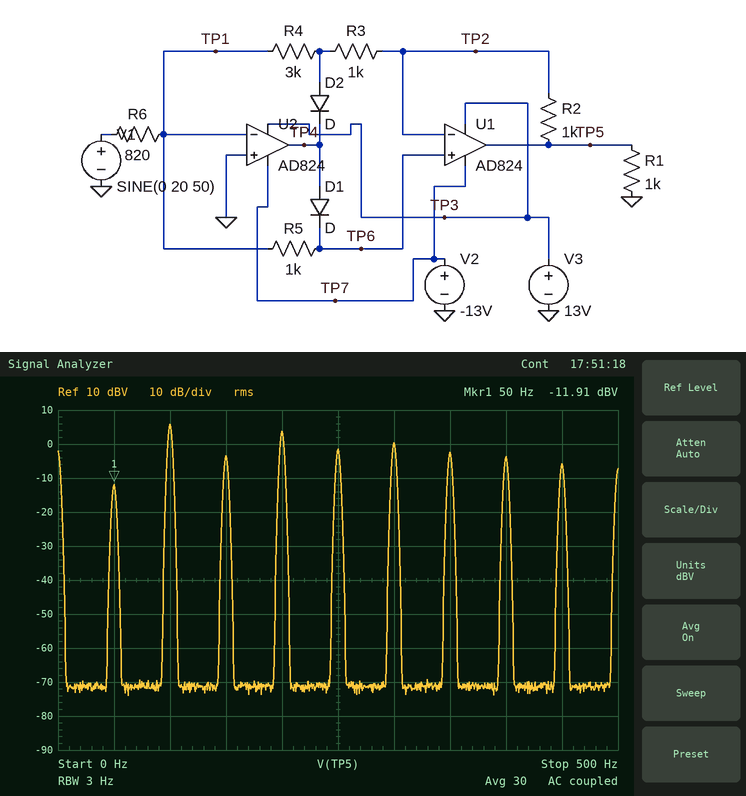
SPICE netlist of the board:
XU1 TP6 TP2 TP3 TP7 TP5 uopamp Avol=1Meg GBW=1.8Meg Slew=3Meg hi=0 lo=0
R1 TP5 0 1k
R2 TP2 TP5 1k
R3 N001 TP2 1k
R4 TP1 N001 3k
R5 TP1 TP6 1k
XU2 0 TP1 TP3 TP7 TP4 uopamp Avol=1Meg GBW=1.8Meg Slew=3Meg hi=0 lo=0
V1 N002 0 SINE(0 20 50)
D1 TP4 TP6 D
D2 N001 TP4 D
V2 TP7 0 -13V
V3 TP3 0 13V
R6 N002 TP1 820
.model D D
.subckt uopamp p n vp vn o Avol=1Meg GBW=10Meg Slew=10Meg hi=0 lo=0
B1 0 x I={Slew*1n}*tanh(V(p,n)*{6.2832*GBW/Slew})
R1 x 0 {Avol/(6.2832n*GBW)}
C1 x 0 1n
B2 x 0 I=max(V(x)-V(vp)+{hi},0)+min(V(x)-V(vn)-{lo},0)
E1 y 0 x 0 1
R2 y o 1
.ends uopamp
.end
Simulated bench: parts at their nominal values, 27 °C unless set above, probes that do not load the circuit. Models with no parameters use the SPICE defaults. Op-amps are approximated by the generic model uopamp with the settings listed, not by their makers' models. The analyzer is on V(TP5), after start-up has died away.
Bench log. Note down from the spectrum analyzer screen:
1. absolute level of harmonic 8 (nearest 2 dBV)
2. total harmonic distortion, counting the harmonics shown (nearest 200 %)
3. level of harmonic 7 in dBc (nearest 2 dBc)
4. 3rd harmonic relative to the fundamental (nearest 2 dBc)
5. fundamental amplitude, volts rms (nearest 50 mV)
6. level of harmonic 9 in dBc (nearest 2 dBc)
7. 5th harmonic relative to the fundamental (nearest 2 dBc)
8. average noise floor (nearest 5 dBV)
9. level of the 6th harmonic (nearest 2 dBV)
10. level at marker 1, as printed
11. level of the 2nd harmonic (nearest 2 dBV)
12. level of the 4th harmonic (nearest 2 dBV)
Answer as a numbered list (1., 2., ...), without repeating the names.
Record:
1. -4 dBV
2. 1200 %
3. 10 dBc
4. 8 dBc
5. 250 mV
6. 6 dBc
7. 10 dBc
8. -70 dBV
9. 0 dBV
10. -11.91 dBV
11. 6 dBV
12. 4 dBV
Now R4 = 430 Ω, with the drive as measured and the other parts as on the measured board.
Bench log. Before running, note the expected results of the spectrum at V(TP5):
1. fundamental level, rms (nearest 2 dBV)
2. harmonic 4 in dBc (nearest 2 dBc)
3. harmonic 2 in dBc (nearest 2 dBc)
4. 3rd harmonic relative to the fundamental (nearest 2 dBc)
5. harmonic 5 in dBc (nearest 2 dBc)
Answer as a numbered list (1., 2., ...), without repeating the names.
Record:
1. 6 dBV
2. -2 dBc
3. 4 dBc
4. -4 dBc
5. -20 dBc
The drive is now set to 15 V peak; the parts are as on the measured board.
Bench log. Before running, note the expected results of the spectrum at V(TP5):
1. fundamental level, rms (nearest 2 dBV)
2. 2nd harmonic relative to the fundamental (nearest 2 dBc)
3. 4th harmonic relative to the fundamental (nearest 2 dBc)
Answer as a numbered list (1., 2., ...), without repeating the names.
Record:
1. -6 dBV
2. 14 dBc
3. 10 dBc
